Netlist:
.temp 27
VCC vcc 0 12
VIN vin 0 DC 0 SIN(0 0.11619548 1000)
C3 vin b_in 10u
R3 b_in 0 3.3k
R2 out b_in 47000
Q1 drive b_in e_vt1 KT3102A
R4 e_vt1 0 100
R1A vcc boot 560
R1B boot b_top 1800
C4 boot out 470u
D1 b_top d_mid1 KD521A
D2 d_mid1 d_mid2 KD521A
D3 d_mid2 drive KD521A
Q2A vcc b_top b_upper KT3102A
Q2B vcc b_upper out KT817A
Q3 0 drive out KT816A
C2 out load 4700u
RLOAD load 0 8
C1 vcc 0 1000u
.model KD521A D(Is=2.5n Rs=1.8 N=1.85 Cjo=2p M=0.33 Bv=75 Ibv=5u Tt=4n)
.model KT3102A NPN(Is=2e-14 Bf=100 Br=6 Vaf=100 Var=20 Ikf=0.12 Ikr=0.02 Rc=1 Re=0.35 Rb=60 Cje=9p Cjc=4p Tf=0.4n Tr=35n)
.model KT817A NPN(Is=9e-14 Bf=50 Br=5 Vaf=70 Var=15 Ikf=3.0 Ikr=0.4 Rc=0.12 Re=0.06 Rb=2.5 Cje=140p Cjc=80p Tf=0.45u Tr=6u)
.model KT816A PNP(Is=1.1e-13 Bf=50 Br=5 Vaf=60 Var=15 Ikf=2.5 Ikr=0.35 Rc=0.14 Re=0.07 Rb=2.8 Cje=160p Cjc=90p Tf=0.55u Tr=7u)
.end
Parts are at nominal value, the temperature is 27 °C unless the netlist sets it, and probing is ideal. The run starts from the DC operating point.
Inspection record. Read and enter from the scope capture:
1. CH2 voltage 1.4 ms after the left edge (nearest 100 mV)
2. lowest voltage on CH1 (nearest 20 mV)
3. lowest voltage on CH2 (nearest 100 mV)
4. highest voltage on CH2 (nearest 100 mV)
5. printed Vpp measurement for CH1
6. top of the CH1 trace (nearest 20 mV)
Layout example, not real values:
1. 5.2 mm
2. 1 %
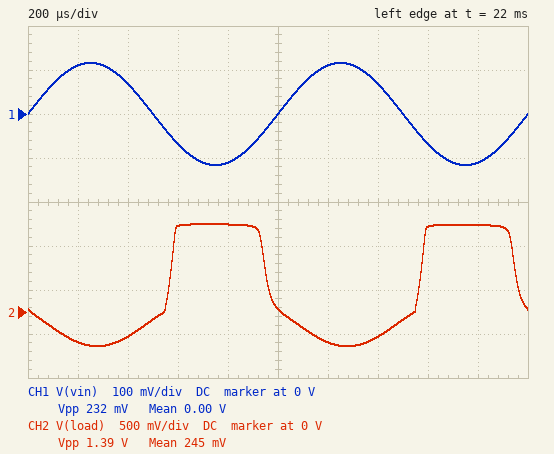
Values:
1. -300 mV
2. -120 mV
3. -400 mV
4. 1.0 V
5. 232 mV
6. 120 mV
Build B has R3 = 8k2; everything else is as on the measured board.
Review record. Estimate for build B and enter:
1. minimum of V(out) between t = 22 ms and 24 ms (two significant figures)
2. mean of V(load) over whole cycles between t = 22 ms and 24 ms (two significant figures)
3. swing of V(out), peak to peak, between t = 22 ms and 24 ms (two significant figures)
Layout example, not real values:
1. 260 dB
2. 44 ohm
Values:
1. 6.5 V
2. 410 mV
3. 4.5 V
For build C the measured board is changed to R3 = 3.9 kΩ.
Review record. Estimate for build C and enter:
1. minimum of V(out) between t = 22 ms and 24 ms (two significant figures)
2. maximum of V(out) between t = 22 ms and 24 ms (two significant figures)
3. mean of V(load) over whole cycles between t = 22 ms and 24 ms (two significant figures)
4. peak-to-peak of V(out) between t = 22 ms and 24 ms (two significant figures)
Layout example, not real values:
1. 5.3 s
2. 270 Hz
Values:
1. 9.2 V
2. 11 V
3. 380 mV
4. 2.0 V
